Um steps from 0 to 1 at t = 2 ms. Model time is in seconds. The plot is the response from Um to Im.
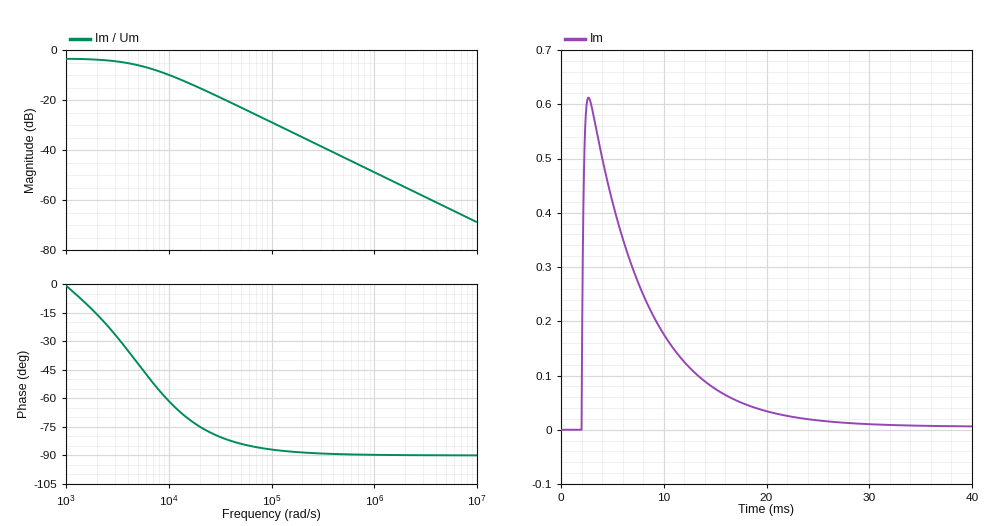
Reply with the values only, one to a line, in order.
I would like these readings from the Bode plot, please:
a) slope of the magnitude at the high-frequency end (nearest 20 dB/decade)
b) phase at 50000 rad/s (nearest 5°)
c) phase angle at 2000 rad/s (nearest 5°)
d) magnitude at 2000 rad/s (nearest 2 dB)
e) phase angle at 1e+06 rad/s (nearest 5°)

-20 dB/decade
-85°
-15°
-4 dB
-90°
